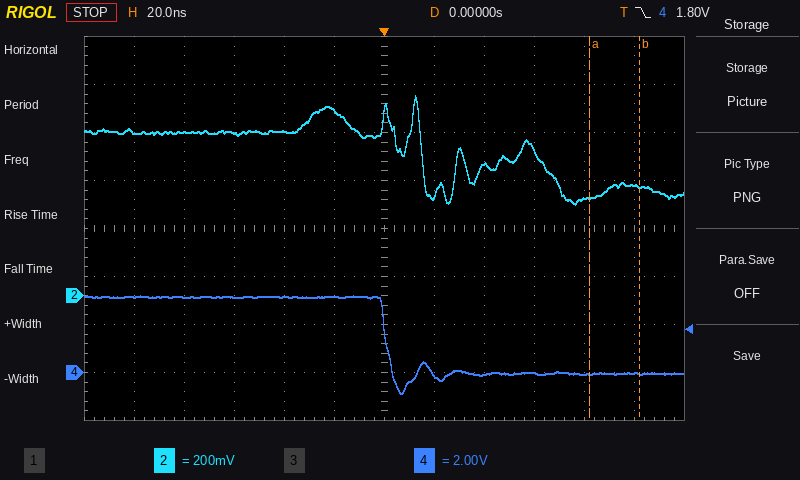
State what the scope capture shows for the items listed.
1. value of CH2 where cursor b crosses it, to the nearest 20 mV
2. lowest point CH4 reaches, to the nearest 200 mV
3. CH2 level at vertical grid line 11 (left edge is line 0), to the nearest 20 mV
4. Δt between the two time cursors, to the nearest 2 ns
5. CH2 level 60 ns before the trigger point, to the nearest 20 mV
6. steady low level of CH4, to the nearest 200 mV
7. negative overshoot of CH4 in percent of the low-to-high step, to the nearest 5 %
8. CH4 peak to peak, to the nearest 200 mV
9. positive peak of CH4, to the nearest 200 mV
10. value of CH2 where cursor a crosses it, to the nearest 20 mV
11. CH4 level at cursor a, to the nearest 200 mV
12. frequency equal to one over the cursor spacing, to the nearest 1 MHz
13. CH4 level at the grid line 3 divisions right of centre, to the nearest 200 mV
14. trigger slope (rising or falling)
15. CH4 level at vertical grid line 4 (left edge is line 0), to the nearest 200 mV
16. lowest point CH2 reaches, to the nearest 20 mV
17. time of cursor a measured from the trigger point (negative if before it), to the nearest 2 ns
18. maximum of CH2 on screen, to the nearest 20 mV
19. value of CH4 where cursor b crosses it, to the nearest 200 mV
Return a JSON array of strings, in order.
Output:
["460 mV", "-800 mV", "460 mV", "20 ns", "680 mV", "0.0 V", "25 %", "4.0 V", "3.2 V", "400 mV", "0.0 V", "50 MHz", "0.0 V", "falling", "3.2 V", "380 mV", "+82 ns", "840 mV", "0.0 V"]
